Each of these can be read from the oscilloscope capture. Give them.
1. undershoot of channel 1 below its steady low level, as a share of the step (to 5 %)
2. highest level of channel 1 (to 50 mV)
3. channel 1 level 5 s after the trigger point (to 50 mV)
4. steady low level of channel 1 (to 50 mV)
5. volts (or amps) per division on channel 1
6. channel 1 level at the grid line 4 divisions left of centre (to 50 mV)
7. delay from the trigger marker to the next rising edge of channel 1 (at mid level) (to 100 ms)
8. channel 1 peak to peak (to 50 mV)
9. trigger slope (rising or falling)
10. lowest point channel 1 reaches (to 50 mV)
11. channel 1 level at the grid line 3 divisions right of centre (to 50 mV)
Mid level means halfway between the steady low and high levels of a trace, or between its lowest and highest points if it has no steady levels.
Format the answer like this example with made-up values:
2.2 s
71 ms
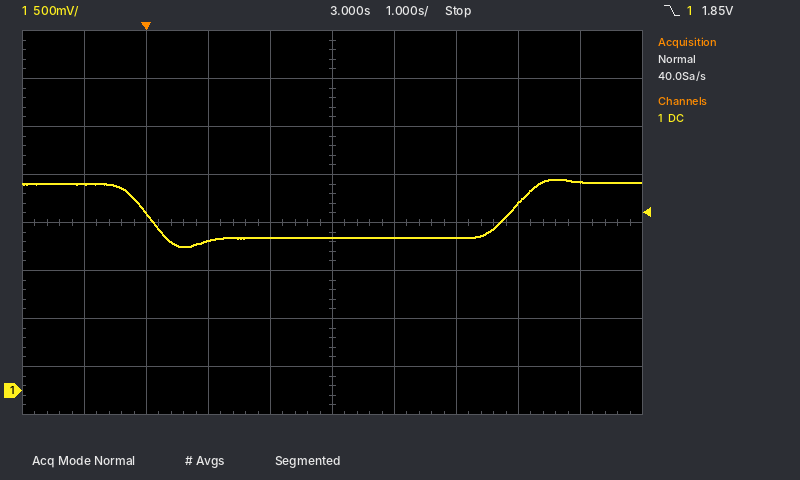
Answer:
15 %
2.20 V
1.60 V
1.60 V
500 mV
2.15 V
5.9 s
700 mV
falling
1.50 V
1.95 V
